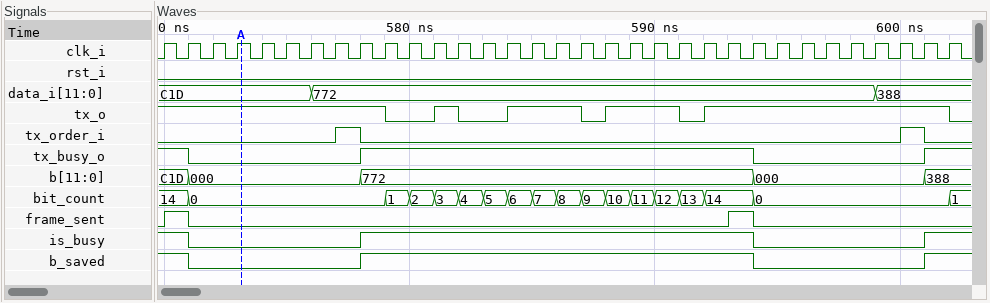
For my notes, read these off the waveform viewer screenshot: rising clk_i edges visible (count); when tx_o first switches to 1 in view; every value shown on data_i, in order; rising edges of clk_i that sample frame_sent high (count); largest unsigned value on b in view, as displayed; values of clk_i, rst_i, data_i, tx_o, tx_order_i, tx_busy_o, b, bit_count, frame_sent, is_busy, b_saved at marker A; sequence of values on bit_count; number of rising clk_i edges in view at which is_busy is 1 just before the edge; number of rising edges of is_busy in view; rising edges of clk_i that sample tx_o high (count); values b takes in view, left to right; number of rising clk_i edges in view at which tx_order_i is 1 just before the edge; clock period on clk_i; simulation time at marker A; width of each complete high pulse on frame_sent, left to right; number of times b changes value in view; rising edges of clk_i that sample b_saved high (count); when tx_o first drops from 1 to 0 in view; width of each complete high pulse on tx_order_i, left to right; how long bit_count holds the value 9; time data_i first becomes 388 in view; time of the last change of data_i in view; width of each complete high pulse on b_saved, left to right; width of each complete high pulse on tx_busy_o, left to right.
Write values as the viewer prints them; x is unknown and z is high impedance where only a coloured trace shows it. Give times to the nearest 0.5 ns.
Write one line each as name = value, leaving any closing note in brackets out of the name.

rising clk_i edges visible = 33
when tx_o first switches to 1 in view = 581 ns
every value shown on data_i, in order = C1D, 772, 388
rising edges of clk_i that sample frame_sent high = 2
largest unsigned value on b in view, as displayed = C1D
values of clk_i, rst_i, data_i, tx_o, tx_order_i, tx_busy_o, b, bit_count, frame_sent, is_busy, b_saved at marker A = clk_i=1, rst_i=0, data_i=C1D, tx_o=1, tx_order_i=0, tx_busy_o=0, b=000, bit_count=0, frame_sent=0, is_busy=0, b_saved=0
sequence of values on bit_count = 14, 0, 1, 2, 3, 4, 5, 6, 7, 8, 9, 10, 11, 12, 13, 14, 0, 1
number of rising clk_i edges in view at which is_busy is 1 just before the edge = 19
number of rising edges of is_busy in view = 2
rising edges of clk_i that sample tx_o high = 27
values b takes in view, left to right = C1D, 000, 772, 000, 388
number of rising clk_i edges in view at which tx_order_i is 1 just before the edge = 2
clock period on clk_i = 1 ns
simulation time at marker A = 573 ns
width of each complete high pulse on frame_sent, left to right = 1 ns, 1 ns
number of times b changes value in view = 4
rising edges of clk_i that sample b_saved high = 19
when tx_o first drops from 1 to 0 in view = 579 ns
width of each complete high pulse on tx_order_i, left to right = 1 ns, 1 ns
how long bit_count holds the value 9 = 1 ns
time data_i first becomes 388 in view = 599 ns
time of the last change of data_i in view = 599 ns
width of each complete high pulse on b_saved, left to right = 16 ns
width of each complete high pulse on tx_busy_o, left to right = 16 ns
